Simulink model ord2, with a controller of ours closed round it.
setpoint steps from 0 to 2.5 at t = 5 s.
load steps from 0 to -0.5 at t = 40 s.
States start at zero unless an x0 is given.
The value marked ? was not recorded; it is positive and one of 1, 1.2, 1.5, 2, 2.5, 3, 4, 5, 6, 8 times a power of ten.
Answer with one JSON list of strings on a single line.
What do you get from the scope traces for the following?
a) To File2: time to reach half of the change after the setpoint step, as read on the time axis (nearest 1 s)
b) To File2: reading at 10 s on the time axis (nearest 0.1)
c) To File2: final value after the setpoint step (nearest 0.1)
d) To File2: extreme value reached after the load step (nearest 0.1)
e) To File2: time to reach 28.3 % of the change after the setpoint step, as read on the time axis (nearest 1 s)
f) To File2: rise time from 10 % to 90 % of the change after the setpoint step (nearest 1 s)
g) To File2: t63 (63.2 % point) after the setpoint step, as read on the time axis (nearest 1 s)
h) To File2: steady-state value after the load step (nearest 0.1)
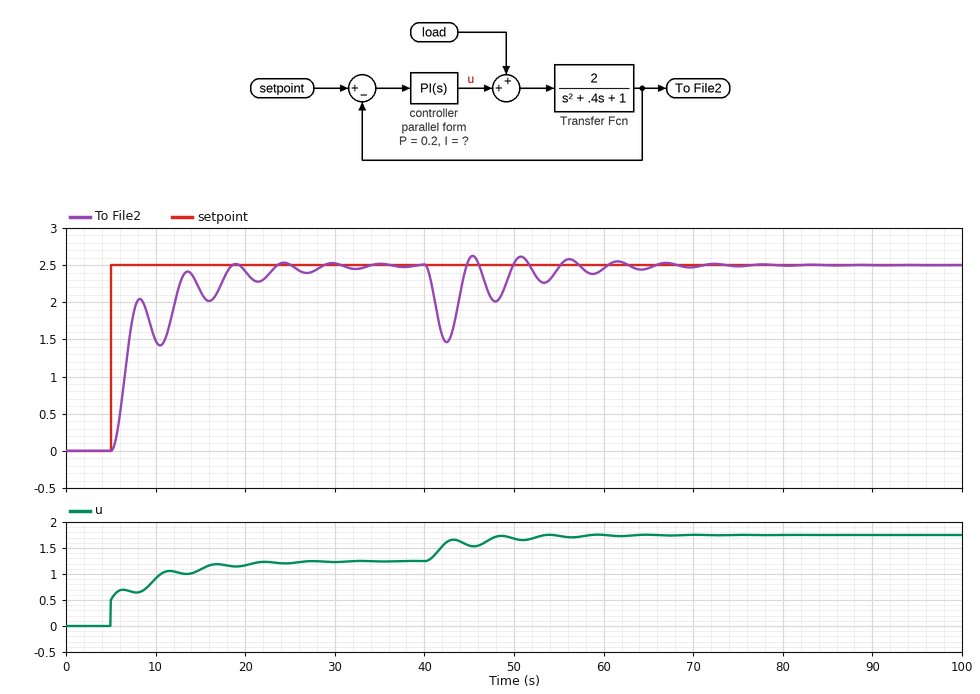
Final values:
["7 s", "1.5", "2.5", "1.5", "6 s", "7 s", "7 s", "2.5"]
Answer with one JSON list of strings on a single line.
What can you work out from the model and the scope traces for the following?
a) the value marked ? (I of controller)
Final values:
["0.12"]
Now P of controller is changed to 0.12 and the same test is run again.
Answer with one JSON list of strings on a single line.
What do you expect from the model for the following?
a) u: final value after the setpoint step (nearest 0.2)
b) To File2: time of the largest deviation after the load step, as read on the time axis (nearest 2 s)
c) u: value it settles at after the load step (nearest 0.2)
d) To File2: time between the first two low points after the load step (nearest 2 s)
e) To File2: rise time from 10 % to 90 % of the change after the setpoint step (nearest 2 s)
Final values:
["1.2", "42 s", "1.8", "6 s", "8 s"]
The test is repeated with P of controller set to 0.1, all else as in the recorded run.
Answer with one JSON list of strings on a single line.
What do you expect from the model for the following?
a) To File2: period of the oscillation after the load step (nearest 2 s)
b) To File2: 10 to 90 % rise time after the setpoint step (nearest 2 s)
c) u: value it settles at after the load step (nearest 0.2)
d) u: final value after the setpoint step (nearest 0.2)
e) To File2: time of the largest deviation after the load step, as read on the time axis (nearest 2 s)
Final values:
["6 s", "8 s", "1.8", "1.2", "42 s"]
